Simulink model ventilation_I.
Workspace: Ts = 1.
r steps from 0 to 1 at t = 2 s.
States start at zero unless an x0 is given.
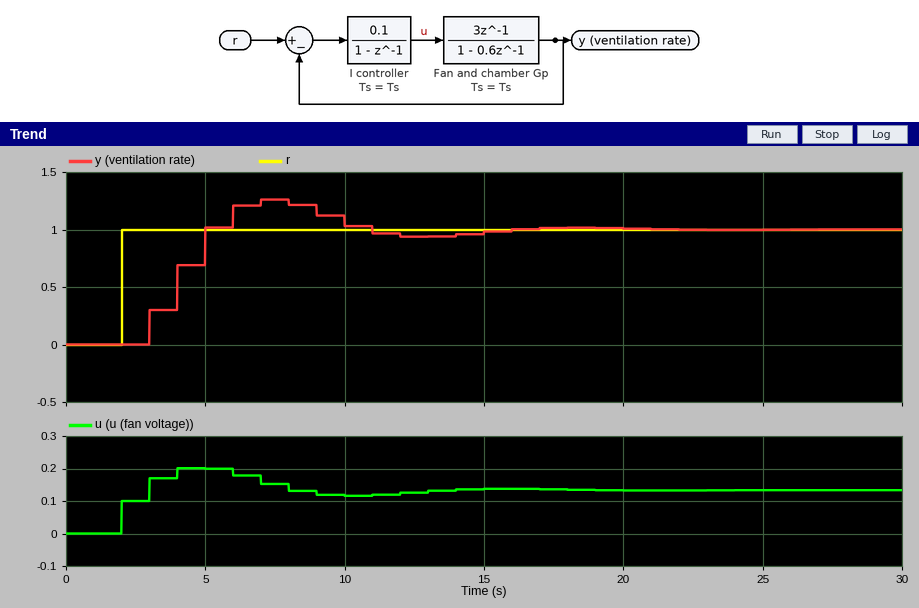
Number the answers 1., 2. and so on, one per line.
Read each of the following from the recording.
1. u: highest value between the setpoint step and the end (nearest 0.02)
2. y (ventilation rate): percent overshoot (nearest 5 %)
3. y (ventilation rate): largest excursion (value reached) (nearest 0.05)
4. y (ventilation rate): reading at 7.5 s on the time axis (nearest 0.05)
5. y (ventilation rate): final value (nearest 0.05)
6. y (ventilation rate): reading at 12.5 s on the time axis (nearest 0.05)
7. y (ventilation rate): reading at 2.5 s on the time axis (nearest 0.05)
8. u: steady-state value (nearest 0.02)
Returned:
1. 0.20
2. 25 %
3. 1.25
4. 1.25
5. 1.00
6. 0.95
7. 0.00
8. 0.14
